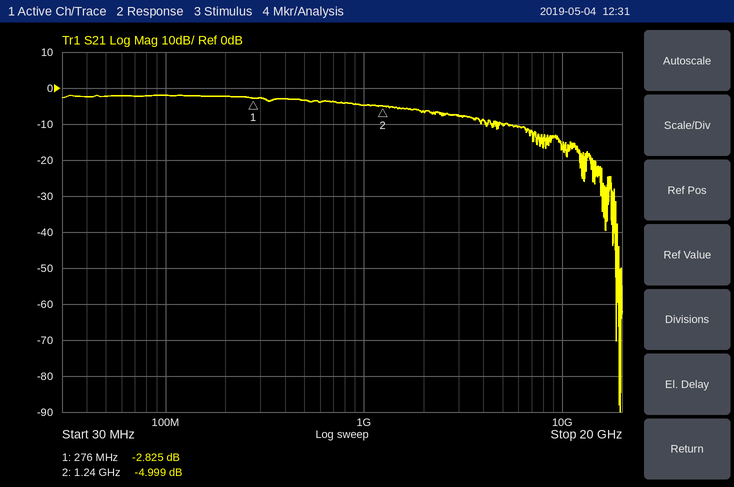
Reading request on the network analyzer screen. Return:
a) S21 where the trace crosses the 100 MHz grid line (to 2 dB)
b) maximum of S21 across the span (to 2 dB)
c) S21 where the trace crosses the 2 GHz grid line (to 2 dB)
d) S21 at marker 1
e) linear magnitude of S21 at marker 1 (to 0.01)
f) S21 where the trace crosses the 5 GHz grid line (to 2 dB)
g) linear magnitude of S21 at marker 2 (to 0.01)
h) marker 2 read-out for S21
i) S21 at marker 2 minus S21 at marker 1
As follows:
-2 dB
-2 dB
-6 dB
-2.825 dB
0.72
-10 dB
0.56
-4.999 dB
-2.174 dB
